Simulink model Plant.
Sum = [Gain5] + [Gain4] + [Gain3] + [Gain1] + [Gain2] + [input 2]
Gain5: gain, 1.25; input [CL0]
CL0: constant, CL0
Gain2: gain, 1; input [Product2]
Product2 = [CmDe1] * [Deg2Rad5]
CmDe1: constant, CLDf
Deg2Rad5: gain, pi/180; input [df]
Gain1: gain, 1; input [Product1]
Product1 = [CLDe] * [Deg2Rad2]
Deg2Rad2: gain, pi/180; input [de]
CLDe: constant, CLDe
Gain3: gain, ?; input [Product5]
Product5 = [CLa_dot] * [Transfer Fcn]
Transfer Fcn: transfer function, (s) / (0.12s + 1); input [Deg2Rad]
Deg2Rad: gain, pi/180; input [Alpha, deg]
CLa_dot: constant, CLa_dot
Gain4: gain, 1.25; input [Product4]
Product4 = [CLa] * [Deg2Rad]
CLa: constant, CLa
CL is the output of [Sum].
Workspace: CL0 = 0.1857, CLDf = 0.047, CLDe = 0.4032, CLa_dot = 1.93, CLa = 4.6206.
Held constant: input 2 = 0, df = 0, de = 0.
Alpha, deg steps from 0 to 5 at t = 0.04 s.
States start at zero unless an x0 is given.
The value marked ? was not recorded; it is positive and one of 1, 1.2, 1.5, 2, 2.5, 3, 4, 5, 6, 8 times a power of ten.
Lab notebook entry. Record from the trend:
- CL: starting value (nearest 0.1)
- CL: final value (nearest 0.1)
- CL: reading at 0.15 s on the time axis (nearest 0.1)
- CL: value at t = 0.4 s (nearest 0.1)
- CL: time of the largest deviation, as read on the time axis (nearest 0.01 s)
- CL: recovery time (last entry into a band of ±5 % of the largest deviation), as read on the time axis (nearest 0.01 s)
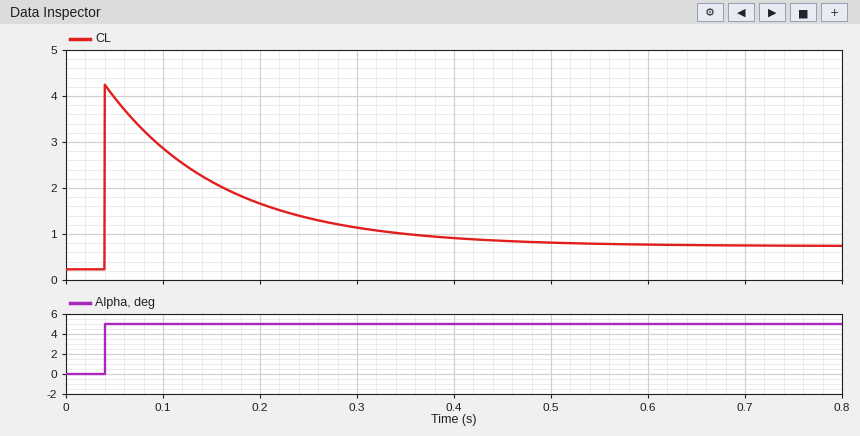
0.2
0.7
2.1
0.9
0.04 s
0.38 s
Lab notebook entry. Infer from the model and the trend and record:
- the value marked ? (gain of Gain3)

2.5
